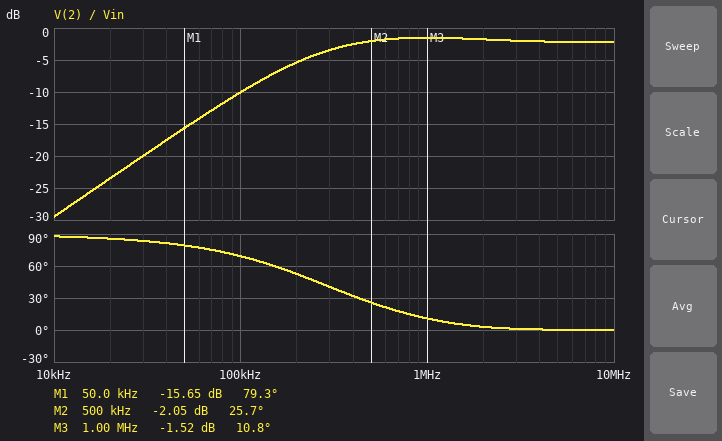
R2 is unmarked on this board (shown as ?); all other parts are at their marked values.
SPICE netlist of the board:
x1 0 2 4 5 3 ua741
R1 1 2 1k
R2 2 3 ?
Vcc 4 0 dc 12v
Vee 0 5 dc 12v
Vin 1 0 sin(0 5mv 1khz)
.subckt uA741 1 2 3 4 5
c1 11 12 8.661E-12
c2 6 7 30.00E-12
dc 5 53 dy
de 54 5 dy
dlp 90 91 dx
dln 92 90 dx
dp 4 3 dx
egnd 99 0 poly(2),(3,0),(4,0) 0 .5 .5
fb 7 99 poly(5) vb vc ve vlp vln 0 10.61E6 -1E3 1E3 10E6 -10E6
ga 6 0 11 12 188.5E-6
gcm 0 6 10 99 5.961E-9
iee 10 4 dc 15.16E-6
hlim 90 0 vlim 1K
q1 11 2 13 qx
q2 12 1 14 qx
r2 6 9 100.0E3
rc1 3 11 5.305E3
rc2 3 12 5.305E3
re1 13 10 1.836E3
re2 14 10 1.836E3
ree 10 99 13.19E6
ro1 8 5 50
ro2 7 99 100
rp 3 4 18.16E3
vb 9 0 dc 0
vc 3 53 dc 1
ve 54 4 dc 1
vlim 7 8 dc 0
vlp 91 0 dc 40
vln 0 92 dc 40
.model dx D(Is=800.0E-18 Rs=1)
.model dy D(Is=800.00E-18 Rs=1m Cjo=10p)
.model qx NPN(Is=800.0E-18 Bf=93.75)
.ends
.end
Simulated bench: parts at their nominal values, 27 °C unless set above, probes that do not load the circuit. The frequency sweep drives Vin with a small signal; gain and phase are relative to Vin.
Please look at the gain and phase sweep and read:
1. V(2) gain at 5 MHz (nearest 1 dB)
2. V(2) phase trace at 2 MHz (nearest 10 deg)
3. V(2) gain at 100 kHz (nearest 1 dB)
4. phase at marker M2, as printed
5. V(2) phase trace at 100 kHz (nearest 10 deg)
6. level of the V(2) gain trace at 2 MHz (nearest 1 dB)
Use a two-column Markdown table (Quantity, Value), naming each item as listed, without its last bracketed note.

| Quantity | Value |
|---|---|
| V(2) gain at 5 MHz | -2 dB |
| V(2) phase trace at 2 MHz | 0 deg |
| V(2) gain at 100 kHz | -10 dB |
| phase at marker M2, as printed | 25.7 deg |
| V(2) phase trace at 100 kHz | 70 deg |
| level of the V(2) gain trace at 2 MHz | -2 dB |
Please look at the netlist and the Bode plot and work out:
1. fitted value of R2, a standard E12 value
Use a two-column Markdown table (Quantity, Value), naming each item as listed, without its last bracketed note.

| Quantity | Value |
|---|---|
| fitted value of R2, a standard E12 value | 3.3 kΩ |
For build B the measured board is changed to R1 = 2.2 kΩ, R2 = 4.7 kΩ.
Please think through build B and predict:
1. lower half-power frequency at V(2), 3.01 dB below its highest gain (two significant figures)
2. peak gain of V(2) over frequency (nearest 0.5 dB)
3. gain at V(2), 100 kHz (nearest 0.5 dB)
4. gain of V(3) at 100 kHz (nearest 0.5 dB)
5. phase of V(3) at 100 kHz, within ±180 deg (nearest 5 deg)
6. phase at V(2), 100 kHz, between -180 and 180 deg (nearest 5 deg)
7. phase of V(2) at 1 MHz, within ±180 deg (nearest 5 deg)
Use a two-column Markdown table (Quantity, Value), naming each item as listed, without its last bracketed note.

| Quantity | Value |
|---|---|
| lower half-power frequency at V(2), 3.01 dB below its highest gain | 320 kHz |
| peak gain of V(2) over frequency | -2.5 dB |
| gain at V(2), 100 kHz | -13.5 dB |
| gain of V(3) at 100 kHz | 6.5 dB |
| phase of V(3) at 100 kHz, within ±180 deg | 160 deg |
| phase at V(2), 100 kHz, between -180 and 180 deg | 75 deg |
| phase of V(2) at 1 MHz, within ±180 deg | 15 deg |
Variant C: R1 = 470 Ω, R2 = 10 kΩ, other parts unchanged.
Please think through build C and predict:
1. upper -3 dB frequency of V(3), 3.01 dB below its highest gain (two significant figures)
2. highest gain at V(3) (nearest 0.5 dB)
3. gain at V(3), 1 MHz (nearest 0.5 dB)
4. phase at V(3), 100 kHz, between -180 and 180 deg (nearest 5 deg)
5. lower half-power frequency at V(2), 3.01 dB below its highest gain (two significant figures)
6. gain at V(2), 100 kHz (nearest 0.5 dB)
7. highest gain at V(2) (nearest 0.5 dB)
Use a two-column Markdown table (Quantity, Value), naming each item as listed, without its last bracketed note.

| Quantity | Value |
|---|---|
| upper -3 dB frequency of V(3), 3.01 dB below its highest gain | 46 kHz |
| highest gain at V(3) | 26.5 dB |
| gain at V(3), 1 MHz | -1.5 dB |
| phase at V(3), 100 kHz, between -180 and 180 deg | 110 deg |
| lower half-power frequency at V(2), 3.01 dB below its highest gain | 45 kHz |
| gain at V(2), 100 kHz | -1.0 dB |
| highest gain at V(2) | 0 dB |
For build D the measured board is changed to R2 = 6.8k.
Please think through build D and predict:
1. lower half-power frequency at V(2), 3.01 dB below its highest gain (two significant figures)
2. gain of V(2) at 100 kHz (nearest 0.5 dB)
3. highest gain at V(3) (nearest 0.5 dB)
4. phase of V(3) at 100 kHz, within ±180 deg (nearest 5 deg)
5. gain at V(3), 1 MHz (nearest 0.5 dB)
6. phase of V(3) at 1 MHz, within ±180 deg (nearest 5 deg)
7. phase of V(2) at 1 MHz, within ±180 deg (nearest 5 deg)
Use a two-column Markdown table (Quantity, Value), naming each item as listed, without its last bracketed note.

| Quantity | Value |
|---|---|
| lower half-power frequency at V(2), 3.01 dB below its highest gain | 130 kHz |
| gain of V(2) at 100 kHz | -5.0 dB |
| highest gain at V(3) | 16.5 dB |
| phase of V(3) at 100 kHz, within ±180 deg | 140 deg |
| gain at V(3), 1 MHz | -2.0 dB |
| phase of V(3) at 1 MHz, within ±180 deg | 65 deg |
| phase of V(2) at 1 MHz, within ±180 deg | 5 deg |
